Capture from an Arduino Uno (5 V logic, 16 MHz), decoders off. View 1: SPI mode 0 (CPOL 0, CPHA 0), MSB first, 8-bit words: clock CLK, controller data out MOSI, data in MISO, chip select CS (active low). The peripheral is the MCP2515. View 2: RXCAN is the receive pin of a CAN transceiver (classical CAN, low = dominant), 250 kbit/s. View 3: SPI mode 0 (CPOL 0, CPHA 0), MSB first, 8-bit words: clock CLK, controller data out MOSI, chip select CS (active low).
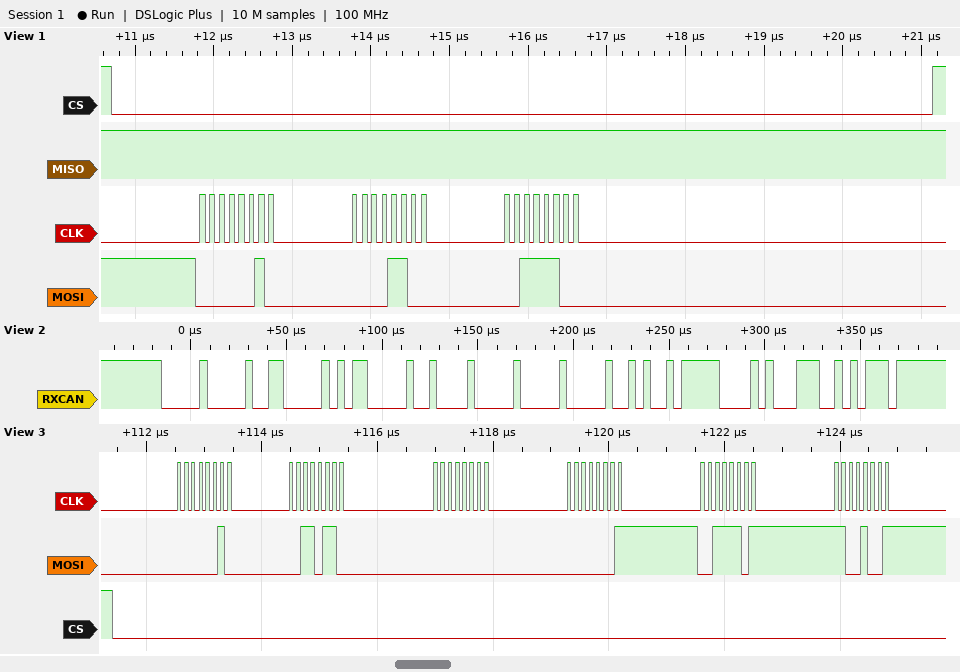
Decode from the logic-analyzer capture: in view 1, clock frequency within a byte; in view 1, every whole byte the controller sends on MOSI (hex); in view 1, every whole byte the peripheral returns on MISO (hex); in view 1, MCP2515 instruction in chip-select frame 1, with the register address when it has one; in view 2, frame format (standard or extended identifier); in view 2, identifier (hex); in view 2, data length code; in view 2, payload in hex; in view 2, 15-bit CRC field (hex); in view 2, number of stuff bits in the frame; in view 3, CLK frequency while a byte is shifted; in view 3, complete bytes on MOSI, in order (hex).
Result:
8 MHz
02 0C 3C
FF FF FF
WRITE 0x0C
extended
0x00000B01
4
00 01 4B E2
0x472B
8
8 MHz
02 36 00 01 3D C9
